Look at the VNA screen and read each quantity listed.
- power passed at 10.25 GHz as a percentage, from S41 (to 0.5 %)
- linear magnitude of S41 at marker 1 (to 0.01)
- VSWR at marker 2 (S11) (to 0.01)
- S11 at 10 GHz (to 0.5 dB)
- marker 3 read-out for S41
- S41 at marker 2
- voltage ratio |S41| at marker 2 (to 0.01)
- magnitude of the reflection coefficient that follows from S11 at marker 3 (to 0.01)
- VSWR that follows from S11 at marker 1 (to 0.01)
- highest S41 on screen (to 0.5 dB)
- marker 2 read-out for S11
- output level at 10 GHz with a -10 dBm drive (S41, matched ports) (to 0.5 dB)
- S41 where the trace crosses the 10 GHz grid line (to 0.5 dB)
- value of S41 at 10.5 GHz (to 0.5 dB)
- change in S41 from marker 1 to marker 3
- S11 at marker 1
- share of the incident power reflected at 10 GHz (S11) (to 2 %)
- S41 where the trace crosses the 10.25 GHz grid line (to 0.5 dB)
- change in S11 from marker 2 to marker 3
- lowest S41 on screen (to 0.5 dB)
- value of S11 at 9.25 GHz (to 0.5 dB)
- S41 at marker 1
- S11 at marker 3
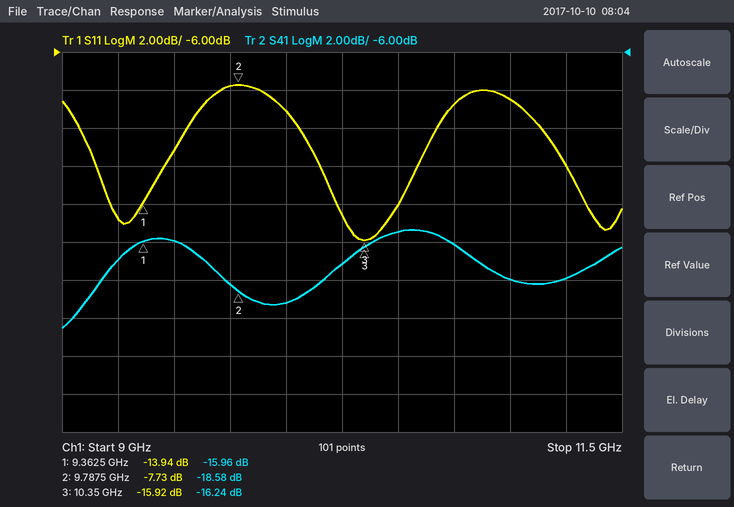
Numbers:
2.0 %
0.16
2.39
-9.0 dB
-16.24 dB
-18.58 dB
0.12
0.16
1.50
-15.5 dB
-7.73 dB
-29.0 dBm
-19.0 dB
-15.5 dB
-0.28 dB
-13.94 dB
12 %
-17.0 dB
-8.19 dB
-20.5 dB
-15.0 dB
-15.96 dB
-15.92 dB
